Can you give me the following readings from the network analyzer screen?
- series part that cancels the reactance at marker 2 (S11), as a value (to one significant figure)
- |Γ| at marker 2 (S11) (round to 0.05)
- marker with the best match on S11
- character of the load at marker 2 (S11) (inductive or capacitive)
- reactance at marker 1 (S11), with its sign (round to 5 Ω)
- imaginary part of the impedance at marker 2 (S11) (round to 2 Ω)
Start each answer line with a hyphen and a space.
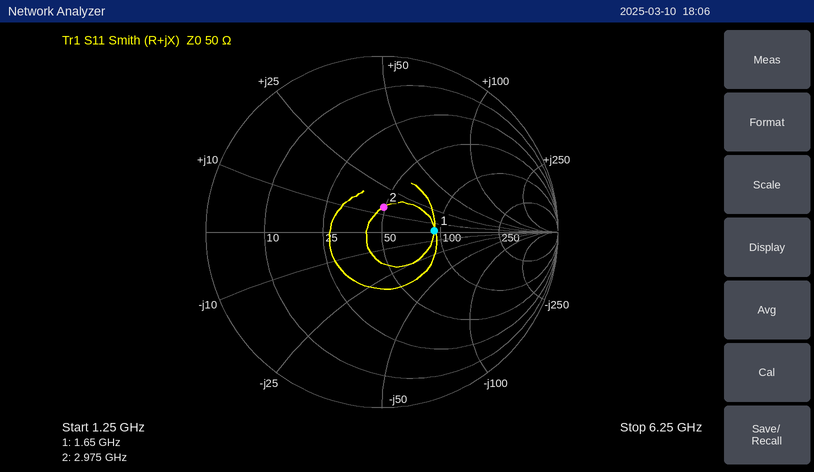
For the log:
- 4 pF
- 0.15
- marker 2
- inductive
- 0 Ω
- +14 Ω
